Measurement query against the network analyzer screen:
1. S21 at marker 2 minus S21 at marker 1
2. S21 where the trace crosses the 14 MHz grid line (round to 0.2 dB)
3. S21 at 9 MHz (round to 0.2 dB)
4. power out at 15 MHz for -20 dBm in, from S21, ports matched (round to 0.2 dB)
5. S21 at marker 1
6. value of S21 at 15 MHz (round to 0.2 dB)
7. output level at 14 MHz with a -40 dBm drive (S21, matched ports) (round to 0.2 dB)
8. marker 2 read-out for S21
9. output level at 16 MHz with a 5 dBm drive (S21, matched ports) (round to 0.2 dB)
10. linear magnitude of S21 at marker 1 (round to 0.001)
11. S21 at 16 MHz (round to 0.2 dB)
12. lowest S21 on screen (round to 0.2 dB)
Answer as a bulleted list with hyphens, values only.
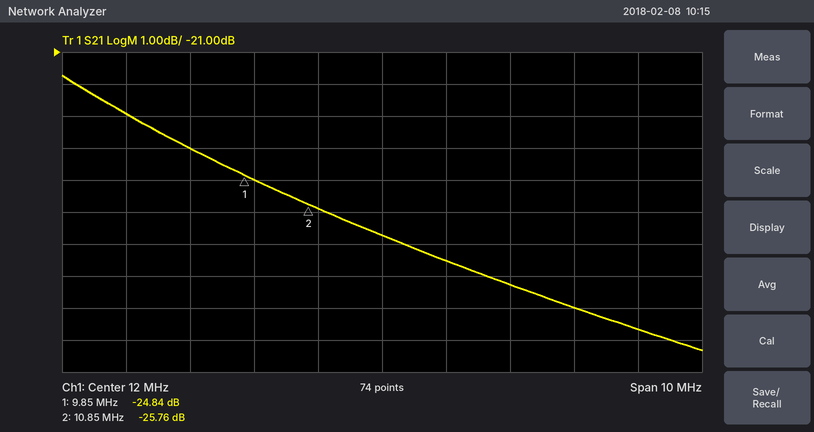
- -0.92 dB
- -28.2 dB
- -24.0 dB
- -49.0 dBm
- -24.84 dB
- -29.0 dB
- -68.2 dBm
- -25.76 dB
- -24.6 dBm
- 0.057
- -29.6 dB
- -30.4 dB
